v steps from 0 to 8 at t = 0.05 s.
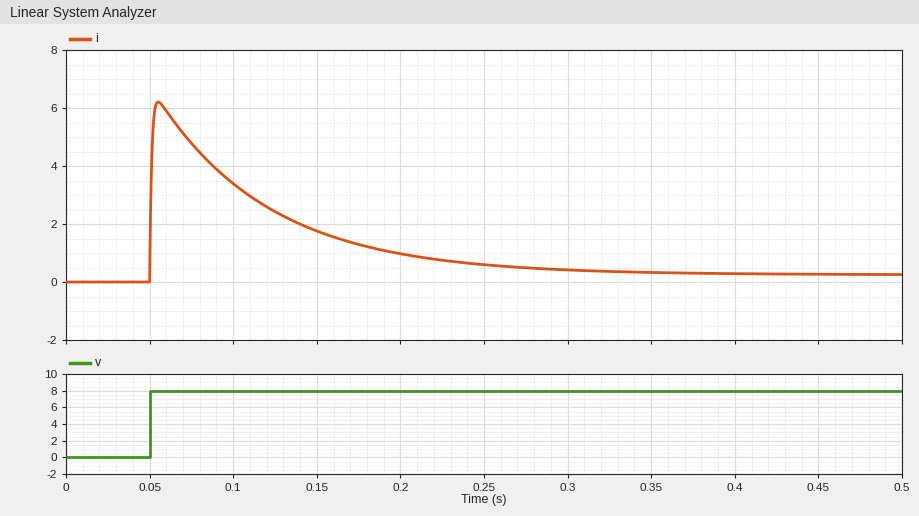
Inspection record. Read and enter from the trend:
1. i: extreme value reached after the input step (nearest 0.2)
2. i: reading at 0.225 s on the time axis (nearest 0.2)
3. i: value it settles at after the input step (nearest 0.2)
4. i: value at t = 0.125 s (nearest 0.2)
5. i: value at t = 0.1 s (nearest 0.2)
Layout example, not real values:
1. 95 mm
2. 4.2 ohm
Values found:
1. 6.2
2. 0.8
3. 0.2
4. 2.4
5. 3.4
